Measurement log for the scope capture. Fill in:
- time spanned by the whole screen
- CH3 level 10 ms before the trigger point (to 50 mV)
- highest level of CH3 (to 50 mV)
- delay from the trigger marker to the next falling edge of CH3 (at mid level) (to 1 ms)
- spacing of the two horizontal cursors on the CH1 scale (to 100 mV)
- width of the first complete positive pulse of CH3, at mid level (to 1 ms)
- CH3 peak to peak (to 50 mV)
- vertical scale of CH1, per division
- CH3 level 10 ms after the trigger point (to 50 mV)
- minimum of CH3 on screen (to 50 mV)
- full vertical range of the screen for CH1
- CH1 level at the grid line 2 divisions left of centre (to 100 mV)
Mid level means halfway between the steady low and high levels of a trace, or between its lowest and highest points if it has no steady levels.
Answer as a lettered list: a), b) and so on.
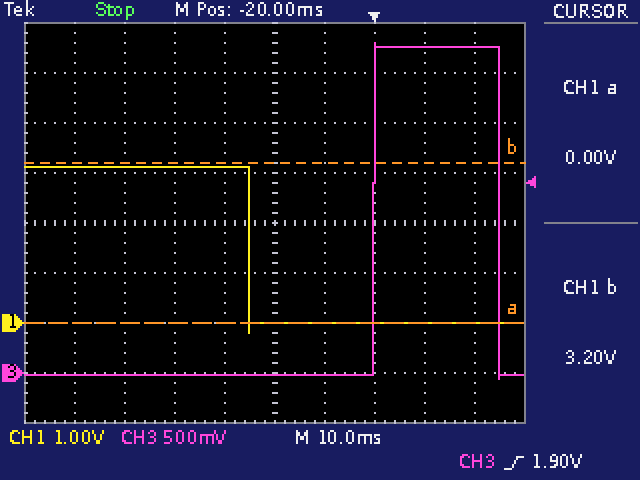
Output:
a) 100 ms
b) 0 mV
c) 3.30 V
d) 25 ms
e) 3.2 V
f) 25 ms
g) 3.35 V
h) 1 V
i) 3.25 V
j) -50 mV
k) 8 V
l) 3.1 V
